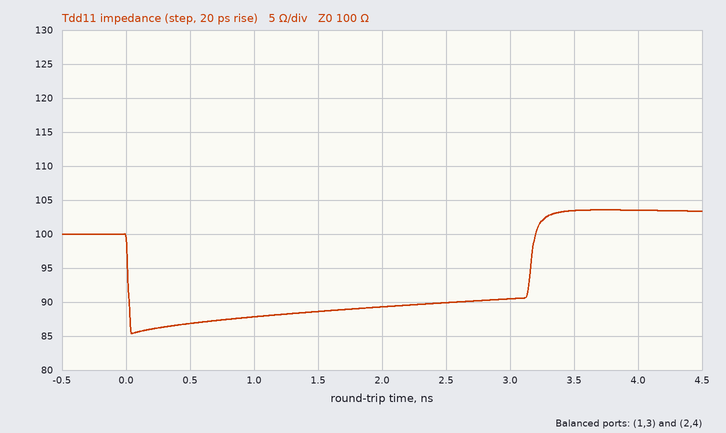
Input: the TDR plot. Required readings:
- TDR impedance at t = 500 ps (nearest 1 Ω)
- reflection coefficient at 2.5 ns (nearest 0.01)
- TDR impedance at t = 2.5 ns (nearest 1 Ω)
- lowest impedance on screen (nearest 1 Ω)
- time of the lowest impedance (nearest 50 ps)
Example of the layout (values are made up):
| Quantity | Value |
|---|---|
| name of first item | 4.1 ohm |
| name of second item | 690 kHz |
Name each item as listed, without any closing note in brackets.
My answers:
| Quantity | Value |
|---|---|
| TDR impedance at t = 500 ps | 87 Ω |
| reflection coefficient at 2.5 ns | -0.05 |
| TDR impedance at t = 2.5 ns | 90 Ω |
| lowest impedance on screen | 85 Ω |
| time of the lowest impedance | 50 ps |
